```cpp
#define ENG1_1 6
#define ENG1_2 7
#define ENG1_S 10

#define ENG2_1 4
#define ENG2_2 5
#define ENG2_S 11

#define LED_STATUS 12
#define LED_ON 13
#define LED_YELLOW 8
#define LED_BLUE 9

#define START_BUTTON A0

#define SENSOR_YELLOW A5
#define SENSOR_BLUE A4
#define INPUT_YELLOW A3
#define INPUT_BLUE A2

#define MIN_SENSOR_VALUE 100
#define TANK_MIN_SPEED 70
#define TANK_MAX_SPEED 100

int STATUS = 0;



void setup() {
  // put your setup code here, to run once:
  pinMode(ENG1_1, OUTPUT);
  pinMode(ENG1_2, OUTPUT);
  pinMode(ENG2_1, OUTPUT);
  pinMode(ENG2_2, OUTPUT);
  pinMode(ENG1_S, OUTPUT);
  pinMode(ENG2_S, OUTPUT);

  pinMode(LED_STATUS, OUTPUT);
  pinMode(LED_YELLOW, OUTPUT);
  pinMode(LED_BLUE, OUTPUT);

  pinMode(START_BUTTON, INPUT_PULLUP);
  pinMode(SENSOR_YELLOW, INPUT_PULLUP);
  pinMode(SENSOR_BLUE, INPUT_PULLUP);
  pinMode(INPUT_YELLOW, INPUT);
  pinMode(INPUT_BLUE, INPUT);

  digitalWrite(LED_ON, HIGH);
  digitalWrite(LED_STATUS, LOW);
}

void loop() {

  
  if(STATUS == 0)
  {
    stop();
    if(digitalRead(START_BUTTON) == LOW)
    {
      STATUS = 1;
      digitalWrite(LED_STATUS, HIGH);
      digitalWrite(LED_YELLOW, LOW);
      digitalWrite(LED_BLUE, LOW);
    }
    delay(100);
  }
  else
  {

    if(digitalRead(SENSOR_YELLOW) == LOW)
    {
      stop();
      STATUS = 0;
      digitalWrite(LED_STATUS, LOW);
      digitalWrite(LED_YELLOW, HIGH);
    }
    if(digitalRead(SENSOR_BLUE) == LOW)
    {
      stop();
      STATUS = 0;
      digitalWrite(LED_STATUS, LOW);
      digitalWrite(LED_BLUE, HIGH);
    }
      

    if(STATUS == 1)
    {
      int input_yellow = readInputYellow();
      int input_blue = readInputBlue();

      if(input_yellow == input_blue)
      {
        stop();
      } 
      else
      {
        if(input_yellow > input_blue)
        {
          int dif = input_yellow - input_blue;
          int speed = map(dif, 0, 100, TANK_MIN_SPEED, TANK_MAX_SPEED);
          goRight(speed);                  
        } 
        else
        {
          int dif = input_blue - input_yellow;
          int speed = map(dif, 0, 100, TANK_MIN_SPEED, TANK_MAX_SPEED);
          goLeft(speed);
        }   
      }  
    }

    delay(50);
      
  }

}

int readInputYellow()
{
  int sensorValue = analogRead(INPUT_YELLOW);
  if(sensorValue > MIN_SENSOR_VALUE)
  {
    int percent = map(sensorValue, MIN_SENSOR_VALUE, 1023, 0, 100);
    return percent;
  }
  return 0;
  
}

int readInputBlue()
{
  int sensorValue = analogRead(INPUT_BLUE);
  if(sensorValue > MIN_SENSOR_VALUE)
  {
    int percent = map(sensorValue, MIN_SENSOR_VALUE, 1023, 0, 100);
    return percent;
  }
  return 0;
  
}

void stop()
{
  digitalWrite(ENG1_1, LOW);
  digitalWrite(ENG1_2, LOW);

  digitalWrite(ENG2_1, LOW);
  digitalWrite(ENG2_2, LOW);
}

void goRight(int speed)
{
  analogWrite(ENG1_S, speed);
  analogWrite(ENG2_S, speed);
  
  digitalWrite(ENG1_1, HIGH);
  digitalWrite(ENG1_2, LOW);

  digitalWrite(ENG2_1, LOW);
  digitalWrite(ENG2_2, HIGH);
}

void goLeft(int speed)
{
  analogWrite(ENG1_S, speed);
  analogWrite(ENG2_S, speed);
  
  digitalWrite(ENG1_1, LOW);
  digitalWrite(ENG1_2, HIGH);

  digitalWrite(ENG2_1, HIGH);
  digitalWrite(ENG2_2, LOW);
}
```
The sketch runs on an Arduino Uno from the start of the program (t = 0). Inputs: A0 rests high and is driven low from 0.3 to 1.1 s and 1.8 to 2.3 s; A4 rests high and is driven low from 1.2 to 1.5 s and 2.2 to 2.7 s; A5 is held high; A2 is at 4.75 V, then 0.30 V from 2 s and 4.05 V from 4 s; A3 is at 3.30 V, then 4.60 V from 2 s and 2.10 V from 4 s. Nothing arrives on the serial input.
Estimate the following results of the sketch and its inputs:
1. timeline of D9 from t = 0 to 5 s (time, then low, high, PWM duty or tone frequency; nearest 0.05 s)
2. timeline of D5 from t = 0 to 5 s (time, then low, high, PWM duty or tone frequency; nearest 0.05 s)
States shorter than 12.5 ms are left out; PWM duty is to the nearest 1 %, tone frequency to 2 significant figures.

0 s low; 1.2 s high; 1.85 s low; 2.2 s high; 2.25 s low; 2.35 s high
0 s low; 2 s high; 2.2 s low
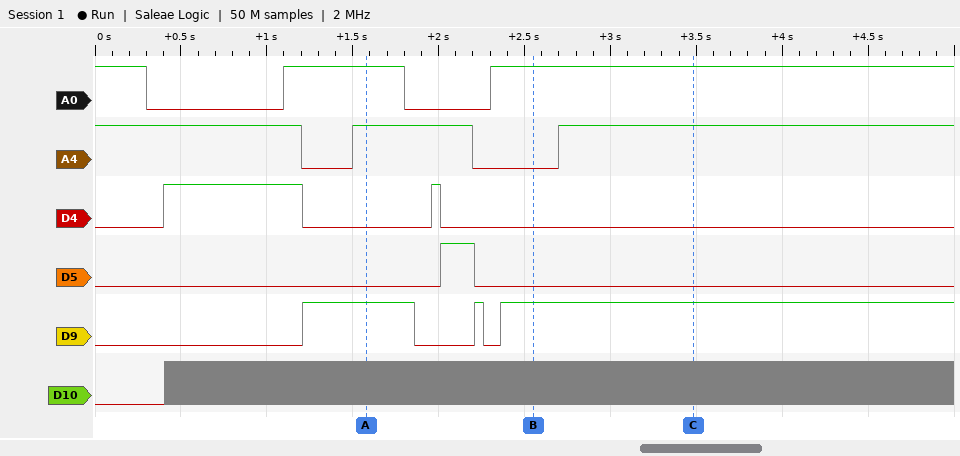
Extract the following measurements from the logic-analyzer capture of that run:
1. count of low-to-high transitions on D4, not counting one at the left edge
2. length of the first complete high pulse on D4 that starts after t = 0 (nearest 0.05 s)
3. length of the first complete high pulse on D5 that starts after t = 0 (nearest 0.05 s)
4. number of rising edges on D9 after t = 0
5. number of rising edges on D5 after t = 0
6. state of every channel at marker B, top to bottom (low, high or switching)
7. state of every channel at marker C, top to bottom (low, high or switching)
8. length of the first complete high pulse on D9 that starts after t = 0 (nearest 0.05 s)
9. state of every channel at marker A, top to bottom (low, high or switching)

2
0.80 s
0.20 s
3
1
A0 high, A4 low, D4 low, D5 low, D9 high, D10 switching
A0 high, A4 high, D4 low, D5 low, D9 high, D10 switching
0.65 s
A0 high, A4 high, D4 low, D5 low, D9 high, D10 switching
